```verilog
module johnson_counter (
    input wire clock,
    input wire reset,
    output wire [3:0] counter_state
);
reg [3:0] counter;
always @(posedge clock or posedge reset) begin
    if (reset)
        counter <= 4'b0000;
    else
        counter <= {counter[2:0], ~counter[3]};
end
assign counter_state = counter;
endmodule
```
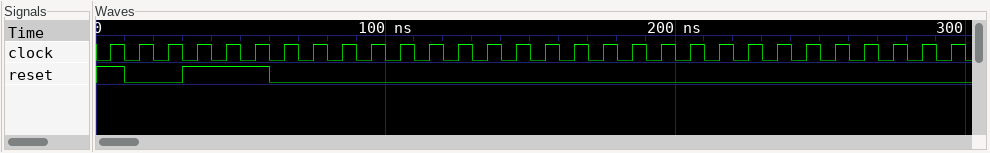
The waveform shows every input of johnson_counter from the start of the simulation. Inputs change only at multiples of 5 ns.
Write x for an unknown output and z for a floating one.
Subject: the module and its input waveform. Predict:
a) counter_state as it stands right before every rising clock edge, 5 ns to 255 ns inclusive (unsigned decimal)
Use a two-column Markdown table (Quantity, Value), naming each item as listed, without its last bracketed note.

| Quantity | Value |
|---|---|
| counter_state as it stands right before every rising clock edge, 5 ns to 255 ns inclusive | 0, 0, 1, 0, 0, 0, 0, 1, 3, 7, 15, 14, 12, 8, 0, 1, 3, 7, 15, 14, 12, 8, 0, 1, 3, 7 |
